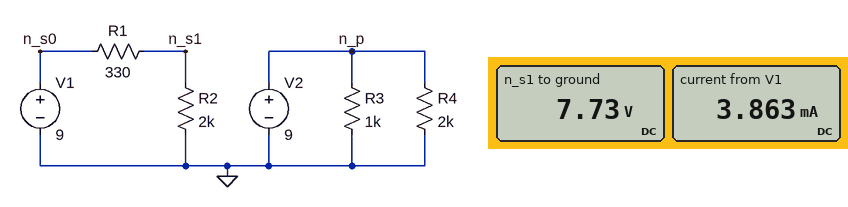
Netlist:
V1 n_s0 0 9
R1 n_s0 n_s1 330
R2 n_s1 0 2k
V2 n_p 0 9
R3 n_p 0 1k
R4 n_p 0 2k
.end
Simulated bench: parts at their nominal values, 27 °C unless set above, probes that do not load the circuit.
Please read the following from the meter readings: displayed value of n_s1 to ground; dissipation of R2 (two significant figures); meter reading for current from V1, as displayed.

7.73 V
30 mW
3.863 mA
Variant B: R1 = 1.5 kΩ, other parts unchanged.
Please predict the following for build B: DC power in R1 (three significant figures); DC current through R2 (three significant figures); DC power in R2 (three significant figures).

9.92 mW
2.57 mA
13.2 mW
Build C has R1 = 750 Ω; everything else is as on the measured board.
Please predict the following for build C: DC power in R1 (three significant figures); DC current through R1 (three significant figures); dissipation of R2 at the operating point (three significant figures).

8.03 mW
3.27 mA
21.4 mW
